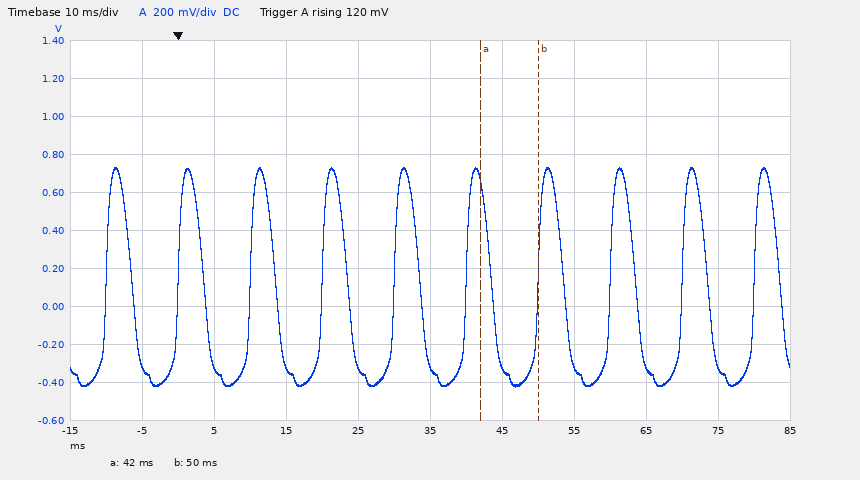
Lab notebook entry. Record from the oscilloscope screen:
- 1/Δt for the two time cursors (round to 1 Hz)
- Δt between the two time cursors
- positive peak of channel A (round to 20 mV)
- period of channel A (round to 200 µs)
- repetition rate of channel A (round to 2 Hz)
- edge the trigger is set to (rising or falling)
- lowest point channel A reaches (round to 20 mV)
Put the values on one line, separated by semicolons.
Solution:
125 Hz; 8 ms; 740 mV; 10.0 ms; 100 Hz; rising; -420 mV
